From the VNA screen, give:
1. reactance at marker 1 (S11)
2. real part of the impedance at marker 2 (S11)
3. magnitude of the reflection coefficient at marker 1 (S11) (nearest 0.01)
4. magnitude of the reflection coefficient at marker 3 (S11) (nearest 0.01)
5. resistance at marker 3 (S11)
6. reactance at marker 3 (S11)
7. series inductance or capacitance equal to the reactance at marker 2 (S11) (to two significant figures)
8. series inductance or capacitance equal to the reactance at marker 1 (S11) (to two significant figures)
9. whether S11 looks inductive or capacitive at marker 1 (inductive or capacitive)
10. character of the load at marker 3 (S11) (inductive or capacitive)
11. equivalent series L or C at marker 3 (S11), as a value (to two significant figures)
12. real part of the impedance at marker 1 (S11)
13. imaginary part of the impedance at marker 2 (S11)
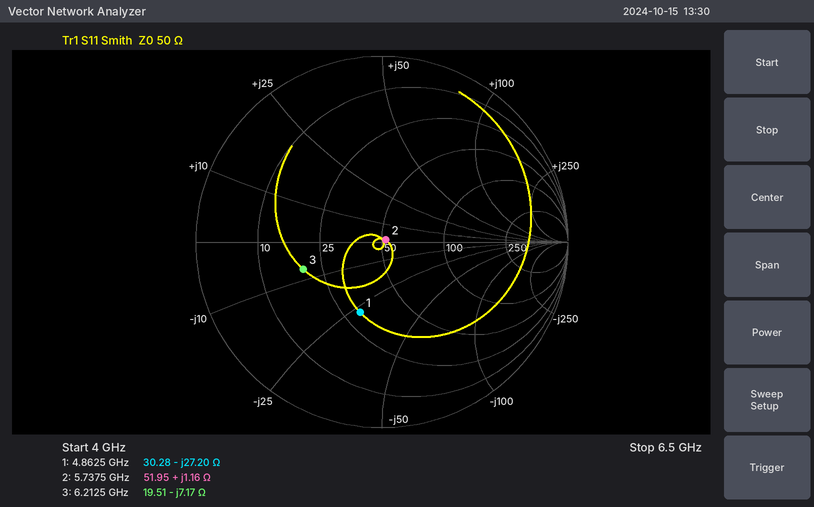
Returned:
-27.20 Ω
51.95 Ω
0.40
0.45
19.51 Ω
-7.17 Ω
32 pH
1.2 pF
capacitive
capacitive
3.6 pF
30.28 Ω
+1.16 Ω
